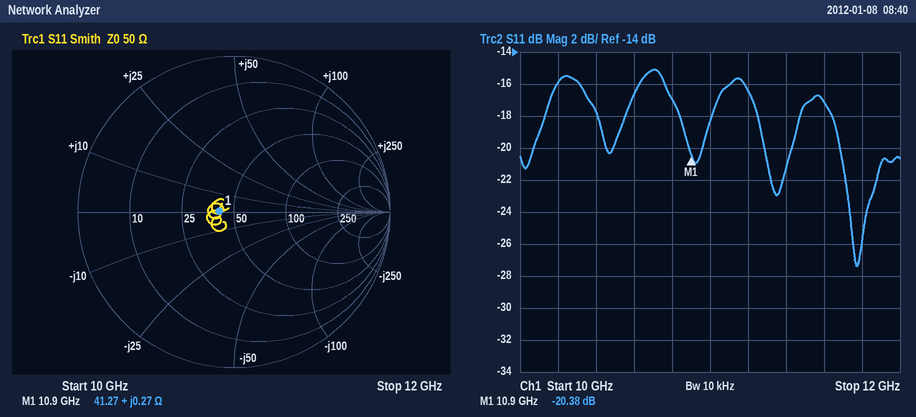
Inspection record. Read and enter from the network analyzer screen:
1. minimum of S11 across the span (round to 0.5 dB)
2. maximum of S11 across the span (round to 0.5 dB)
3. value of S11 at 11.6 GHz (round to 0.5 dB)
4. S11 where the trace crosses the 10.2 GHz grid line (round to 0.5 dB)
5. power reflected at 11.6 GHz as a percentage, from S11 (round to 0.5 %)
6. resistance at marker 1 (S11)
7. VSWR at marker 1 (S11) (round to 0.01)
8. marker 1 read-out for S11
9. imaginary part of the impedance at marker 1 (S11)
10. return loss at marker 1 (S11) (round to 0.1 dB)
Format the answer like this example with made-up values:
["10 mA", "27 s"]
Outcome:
["-27.5 dB", "-15.0 dB", "-17.0 dB", "-16.0 dB", "2.0 %", "41.27 Ω", "1.21", "-20.38 dB", "+0.27 Ω", "20.4 dB"]
